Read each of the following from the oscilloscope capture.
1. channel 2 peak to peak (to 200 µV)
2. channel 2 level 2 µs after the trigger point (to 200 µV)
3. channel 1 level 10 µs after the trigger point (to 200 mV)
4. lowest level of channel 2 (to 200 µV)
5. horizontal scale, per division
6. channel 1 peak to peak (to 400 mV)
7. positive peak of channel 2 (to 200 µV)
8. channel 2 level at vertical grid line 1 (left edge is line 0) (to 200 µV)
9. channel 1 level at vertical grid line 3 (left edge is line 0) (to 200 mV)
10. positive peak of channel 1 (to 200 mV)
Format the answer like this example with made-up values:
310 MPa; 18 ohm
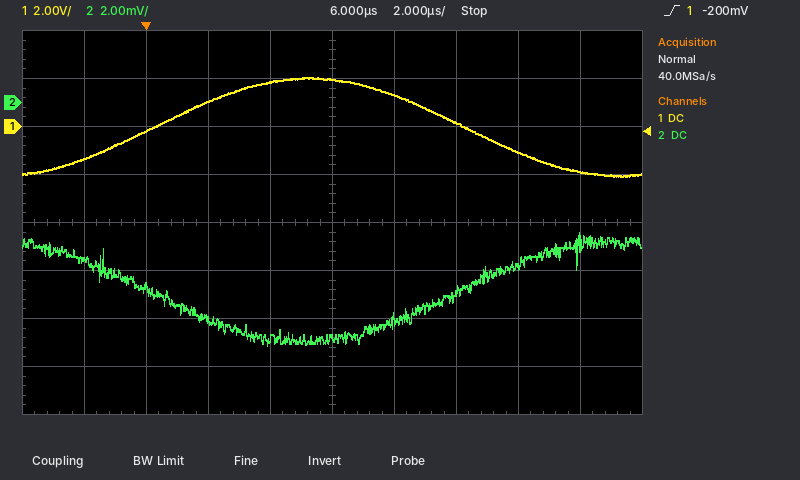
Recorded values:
4.8 mV; -9.0 mV; 200 mV; -10.2 mV; 2 µs; 4.0 V; -5.4 mV; -6.6 mV; 1.0 V; 2.0 V
